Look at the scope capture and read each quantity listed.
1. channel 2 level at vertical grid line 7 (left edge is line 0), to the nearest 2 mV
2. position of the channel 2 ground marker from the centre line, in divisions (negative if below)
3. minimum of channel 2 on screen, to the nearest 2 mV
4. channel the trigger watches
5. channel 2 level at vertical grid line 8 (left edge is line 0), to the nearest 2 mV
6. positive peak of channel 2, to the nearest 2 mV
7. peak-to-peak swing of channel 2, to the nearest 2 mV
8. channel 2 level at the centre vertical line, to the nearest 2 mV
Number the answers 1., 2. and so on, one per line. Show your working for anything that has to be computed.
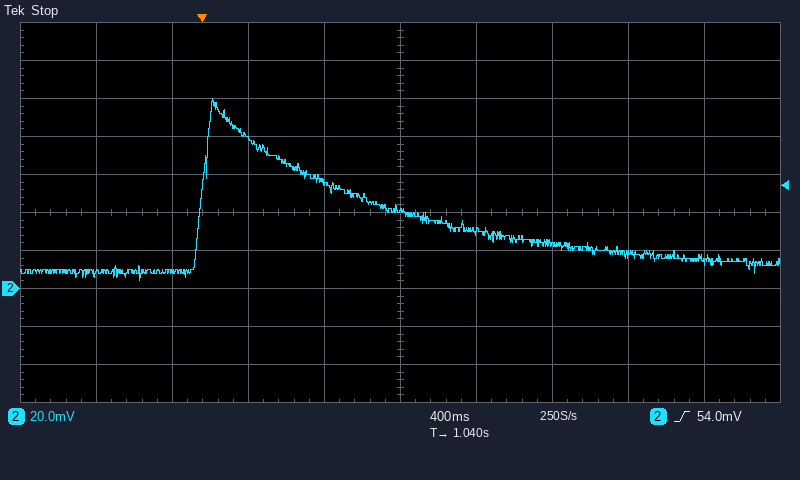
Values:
1. 24 mV
2. -2.0 div
3. 4 mV
4. channel 2
5. 18 mV
6. 100 mV
7. 100 mV − (4 mV) = 96 mV
8. 42 mV
